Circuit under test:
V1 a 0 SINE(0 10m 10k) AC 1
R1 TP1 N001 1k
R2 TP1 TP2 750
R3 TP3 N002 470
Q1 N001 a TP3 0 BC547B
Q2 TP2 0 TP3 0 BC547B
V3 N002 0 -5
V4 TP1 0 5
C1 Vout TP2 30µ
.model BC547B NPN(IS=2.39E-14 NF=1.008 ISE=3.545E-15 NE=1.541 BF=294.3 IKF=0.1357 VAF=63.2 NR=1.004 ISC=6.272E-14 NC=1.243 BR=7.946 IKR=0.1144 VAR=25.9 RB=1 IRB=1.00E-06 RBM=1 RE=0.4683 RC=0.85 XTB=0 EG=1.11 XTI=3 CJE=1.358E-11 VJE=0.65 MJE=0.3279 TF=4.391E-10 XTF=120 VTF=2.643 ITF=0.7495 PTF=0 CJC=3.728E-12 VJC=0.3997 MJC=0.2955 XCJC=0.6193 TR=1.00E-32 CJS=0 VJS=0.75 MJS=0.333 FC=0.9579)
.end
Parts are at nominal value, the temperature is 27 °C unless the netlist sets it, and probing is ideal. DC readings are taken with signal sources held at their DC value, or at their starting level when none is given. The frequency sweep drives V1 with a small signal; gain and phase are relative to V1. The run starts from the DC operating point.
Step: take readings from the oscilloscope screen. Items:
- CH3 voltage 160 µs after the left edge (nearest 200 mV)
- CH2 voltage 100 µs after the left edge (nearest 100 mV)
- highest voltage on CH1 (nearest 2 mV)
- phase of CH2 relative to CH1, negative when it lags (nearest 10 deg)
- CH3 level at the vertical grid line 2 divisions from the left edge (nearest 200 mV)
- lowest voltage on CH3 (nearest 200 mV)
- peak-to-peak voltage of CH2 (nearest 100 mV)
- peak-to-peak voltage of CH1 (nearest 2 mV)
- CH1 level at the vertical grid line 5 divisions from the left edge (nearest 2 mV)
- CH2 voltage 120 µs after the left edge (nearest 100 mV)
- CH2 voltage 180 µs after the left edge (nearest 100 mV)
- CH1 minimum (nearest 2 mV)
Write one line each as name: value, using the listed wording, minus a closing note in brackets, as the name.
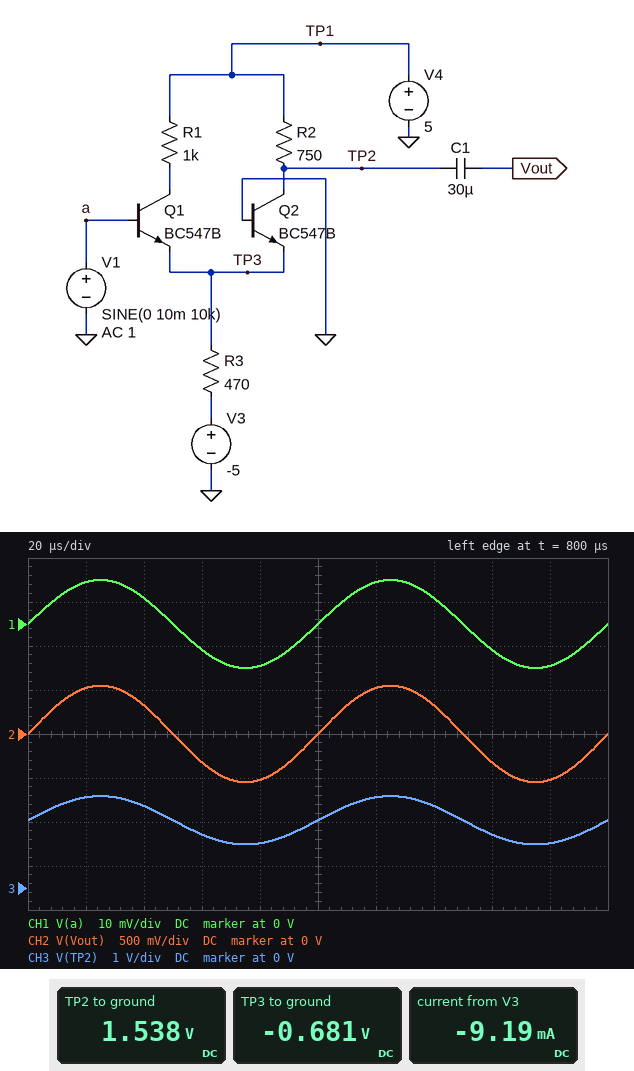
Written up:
CH3 voltage 160 µs after the left edge: 1.2 V
CH2 voltage 100 µs after the left edge: 0 V
highest voltage on CH1: 10 mV
phase of CH2 relative to CH1, negative when it lags: 0 deg
CH3 level at the vertical grid line 2 divisions from the left edge: 1.8 V
lowest voltage on CH3: 1.0 V
peak-to-peak voltage of CH2: 1.1 V
peak-to-peak voltage of CH1: 20 mV
CH1 level at the vertical grid line 5 divisions from the left edge: 0 V
CH2 voltage 120 µs after the left edge: 500 mV
CH2 voltage 180 µs after the left edge: -500 mV
CH1 minimum: -10 mV
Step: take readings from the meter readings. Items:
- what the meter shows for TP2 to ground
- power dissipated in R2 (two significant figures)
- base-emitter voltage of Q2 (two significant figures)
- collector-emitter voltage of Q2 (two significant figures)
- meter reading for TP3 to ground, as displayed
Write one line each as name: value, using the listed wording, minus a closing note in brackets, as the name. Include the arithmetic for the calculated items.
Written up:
what the meter shows for TP2 to ground: 1.538 V
power dissipated in R2: (5 V - 1.538 V)^2 / 750 Ω = 16 mW
base-emitter voltage of Q2: 0 V - (-681 mV) = 680 mV
collector-emitter voltage of Q2: 1.538 V - (-681 mV) = 2.2 V
meter reading for TP3 to ground, as displayed: -0.681 V
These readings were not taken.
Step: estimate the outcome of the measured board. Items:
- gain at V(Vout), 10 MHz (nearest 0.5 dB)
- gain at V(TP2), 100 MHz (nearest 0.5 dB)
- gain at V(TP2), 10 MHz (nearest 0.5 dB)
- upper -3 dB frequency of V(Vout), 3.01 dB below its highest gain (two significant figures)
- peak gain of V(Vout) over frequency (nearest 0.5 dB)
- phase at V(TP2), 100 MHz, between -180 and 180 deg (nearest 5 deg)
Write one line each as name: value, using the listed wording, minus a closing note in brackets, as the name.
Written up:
gain at V(Vout), 10 MHz: 35.0 dB
gain at V(TP2), 100 MHz: 31.0 dB
gain at V(TP2), 10 MHz: 35.0 dB
upper -3 dB frequency of V(Vout), 3.01 dB below its highest gain: 86 MHz
peak gain of V(Vout) over frequency: 35.0 dB
phase at V(TP2), 100 MHz, between -180 and 180 deg: -55 deg
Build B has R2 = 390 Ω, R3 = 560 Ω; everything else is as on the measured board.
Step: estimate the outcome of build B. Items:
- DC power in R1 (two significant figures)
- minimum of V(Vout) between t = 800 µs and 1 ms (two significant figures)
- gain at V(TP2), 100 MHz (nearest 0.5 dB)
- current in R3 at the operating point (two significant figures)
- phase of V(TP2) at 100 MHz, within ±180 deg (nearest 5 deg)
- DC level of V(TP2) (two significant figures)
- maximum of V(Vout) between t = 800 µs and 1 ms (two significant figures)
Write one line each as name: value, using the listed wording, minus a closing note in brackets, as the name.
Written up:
DC power in R1: 14 mW
minimum of V(Vout) between t = 800 µs and 1 ms: -250 mV
gain at V(TP2), 100 MHz: 27.0 dB
current in R3 at the operating point: 7.7 mA
phase of V(TP2) at 100 MHz, within ±180 deg: -30 deg
DC level of V(TP2): 3.5 V
maximum of V(Vout) between t = 800 µs and 1 ms: 250 mV
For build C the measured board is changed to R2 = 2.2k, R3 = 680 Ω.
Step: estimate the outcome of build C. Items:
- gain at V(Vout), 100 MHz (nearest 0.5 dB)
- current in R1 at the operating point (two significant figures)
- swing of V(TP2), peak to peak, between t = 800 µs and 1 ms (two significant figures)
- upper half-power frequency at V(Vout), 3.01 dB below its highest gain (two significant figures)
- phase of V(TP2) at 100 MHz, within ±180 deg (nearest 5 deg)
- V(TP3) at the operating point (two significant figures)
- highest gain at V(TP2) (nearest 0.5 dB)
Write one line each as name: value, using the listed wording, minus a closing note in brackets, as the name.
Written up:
gain at V(Vout), 100 MHz: 2.0 dB
current in R1 at the operating point: 3.6 mA
swing of V(TP2), peak to peak, between t = 800 µs and 1 ms: 89 mV
upper half-power frequency at V(Vout), 3.01 dB below its highest gain: 48 MHz
phase of V(TP2) at 100 MHz, within ±180 deg: -60 deg
V(TP3) at the operating point: -670 mV
highest gain at V(TP2): 9.0 dB
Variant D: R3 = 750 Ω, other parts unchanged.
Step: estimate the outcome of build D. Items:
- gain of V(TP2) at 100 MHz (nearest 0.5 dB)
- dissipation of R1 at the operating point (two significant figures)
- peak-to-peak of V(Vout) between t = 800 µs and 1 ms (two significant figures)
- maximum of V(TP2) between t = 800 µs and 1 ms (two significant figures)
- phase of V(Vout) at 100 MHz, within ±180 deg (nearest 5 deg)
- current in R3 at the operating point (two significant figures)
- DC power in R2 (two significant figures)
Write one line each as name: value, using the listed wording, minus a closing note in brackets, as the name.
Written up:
gain of V(TP2) at 100 MHz: 28.5 dB
dissipation of R1 at the operating point: 8.2 mW
peak-to-peak of V(Vout) between t = 800 µs and 1 ms: 730 mV
maximum of V(TP2) between t = 800 µs and 1 ms: 3.2 V
phase of V(Vout) at 100 MHz, within ±180 deg: -50 deg
current in R3 at the operating point: 5.8 mA
DC power in R2: 6.3 mW
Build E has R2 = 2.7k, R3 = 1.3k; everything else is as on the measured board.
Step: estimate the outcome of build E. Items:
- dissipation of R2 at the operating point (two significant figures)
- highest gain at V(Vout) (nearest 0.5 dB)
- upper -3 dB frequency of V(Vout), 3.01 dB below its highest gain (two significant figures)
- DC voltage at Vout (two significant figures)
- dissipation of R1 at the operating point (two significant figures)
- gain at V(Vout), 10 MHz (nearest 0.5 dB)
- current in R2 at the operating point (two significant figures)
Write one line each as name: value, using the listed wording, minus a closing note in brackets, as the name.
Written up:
dissipation of R2 at the operating point: 7.2 mW
highest gain at V(Vout): 38.0 dB
upper -3 dB frequency of V(Vout), 3.01 dB below its highest gain: 21 MHz
DC voltage at Vout: 590 mV
dissipation of R1 at the operating point: 2.9 mW
gain at V(Vout), 10 MHz: 37.0 dB
current in R2 at the operating point: 1.6 mA
